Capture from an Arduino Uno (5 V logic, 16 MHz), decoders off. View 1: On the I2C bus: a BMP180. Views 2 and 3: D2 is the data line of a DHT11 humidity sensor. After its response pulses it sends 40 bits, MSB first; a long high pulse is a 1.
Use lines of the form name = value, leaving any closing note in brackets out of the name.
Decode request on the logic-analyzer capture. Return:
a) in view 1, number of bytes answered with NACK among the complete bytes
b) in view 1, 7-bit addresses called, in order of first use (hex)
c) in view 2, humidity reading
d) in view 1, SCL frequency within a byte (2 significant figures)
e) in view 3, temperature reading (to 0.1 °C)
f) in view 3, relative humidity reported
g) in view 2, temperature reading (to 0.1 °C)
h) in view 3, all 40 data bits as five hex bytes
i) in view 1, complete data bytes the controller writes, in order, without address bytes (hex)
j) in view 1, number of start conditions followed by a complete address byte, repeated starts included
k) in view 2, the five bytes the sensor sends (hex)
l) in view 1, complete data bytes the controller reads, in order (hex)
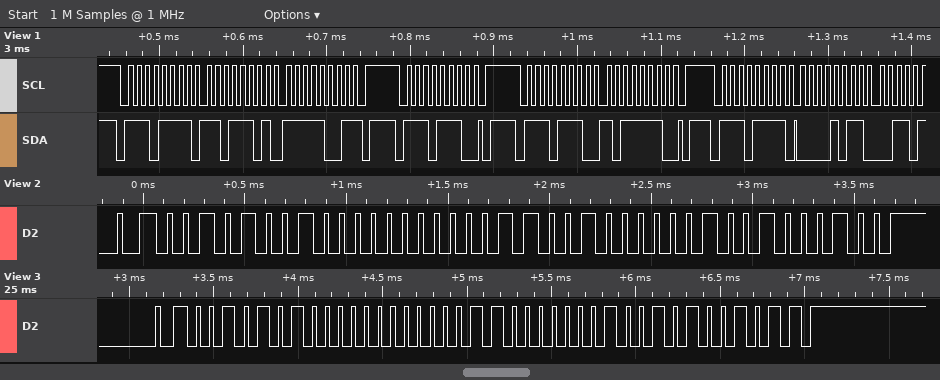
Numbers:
in view 1, number of bytes answered with NACK among the complete bytes = 1
in view 1, 7-bit addresses called, in order of first use = 0x77
in view 2, humidity reading = 41 %
in view 1, SCL frequency within a byte = 100 kHz
in view 3, temperature reading = 24.9 °C
in view 3, relative humidity reported = 42 %
in view 2, temperature reading = 25.2 °C
in view 3, all 40 data bits as five hex bytes = 2A 00 18 09 4B
in view 1, complete data bytes the controller writes, in order, without address bytes = BE
in view 1, number of start conditions followed by a complete address byte, repeated starts included = 4
in view 2, the five bytes the sensor sends = 29 00 19 02 44
in view 1, complete data bytes the controller reads, in order = DD F9 0B
